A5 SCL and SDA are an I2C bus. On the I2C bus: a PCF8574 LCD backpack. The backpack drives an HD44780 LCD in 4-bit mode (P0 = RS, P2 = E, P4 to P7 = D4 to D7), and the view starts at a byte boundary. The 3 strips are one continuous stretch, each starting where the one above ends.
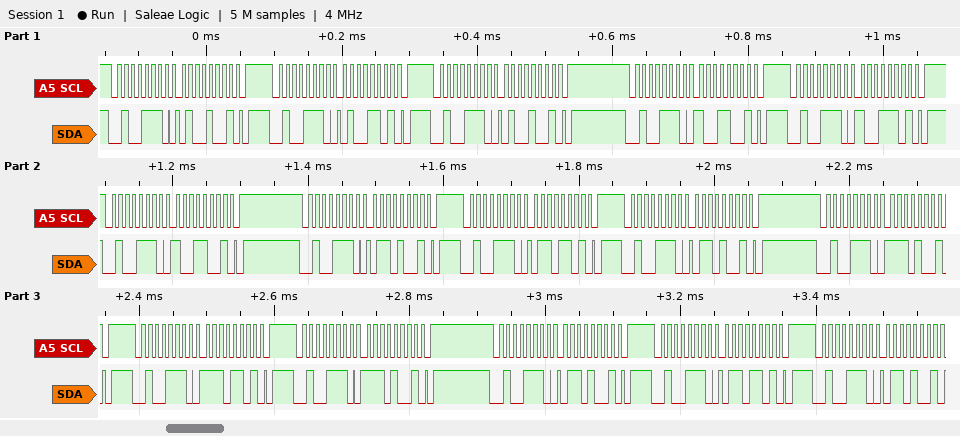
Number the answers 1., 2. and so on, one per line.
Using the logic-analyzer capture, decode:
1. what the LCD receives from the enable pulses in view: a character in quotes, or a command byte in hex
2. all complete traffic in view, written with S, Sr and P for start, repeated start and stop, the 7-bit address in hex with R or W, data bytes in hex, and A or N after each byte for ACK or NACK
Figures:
1. 'I' 'n'
2. S 27W A 49 A P S 27W A 4D A P S 27W A 49 A P S 27W A 99 A P S 27W A 9D A P S 27W A 99 A P S 27W A 69 A P S 27W A 6D A P S 27W A 69 A P S 27W A E9 A P S 27W A ED A P S 27W A E9 A P S 27W A 69 A P S 27W A 6D A P S 27W A 69 A
